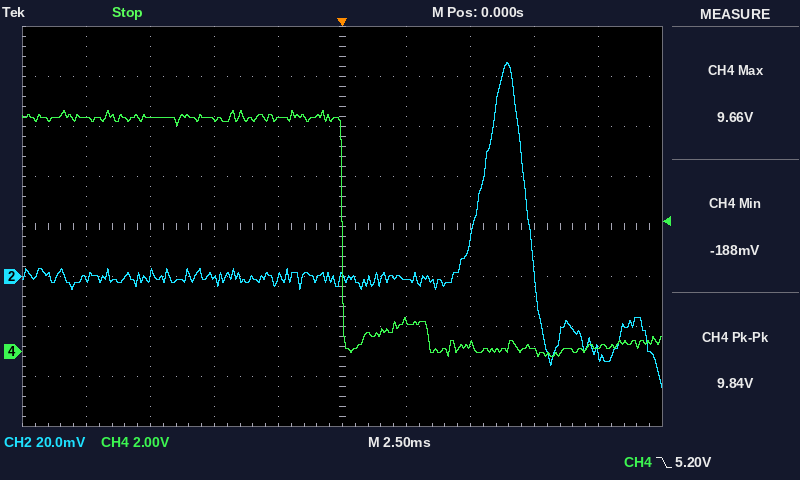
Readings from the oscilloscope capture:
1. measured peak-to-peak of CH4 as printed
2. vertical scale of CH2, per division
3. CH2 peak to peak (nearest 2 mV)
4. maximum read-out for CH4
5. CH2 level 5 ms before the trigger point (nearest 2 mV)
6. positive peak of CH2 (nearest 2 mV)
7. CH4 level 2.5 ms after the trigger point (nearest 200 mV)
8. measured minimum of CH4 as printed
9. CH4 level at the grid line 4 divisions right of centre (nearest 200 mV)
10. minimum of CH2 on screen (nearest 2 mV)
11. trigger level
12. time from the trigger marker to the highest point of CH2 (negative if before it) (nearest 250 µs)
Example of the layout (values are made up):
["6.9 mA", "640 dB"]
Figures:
["9.84 V", "20 mV", "130 mV", "9.66 V", "0 mV", "86 mV", "1.2 V", "-188 mV", "200 mV", "-44 mV", "5.20 V", "+6.50 ms"]
